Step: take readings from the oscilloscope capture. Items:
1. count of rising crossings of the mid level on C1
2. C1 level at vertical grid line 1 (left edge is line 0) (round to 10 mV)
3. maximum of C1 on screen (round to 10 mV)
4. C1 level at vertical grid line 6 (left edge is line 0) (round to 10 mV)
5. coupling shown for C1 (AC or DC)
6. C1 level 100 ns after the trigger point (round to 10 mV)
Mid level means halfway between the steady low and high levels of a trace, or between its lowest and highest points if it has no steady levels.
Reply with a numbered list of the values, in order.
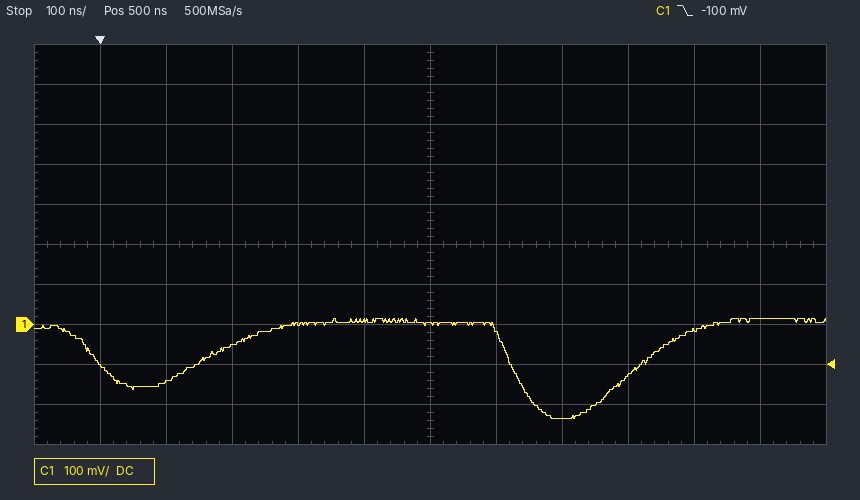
1. 2
2. -100 mV
3. 10 mV
4. 0 mV
5. DC
6. -140 mV
